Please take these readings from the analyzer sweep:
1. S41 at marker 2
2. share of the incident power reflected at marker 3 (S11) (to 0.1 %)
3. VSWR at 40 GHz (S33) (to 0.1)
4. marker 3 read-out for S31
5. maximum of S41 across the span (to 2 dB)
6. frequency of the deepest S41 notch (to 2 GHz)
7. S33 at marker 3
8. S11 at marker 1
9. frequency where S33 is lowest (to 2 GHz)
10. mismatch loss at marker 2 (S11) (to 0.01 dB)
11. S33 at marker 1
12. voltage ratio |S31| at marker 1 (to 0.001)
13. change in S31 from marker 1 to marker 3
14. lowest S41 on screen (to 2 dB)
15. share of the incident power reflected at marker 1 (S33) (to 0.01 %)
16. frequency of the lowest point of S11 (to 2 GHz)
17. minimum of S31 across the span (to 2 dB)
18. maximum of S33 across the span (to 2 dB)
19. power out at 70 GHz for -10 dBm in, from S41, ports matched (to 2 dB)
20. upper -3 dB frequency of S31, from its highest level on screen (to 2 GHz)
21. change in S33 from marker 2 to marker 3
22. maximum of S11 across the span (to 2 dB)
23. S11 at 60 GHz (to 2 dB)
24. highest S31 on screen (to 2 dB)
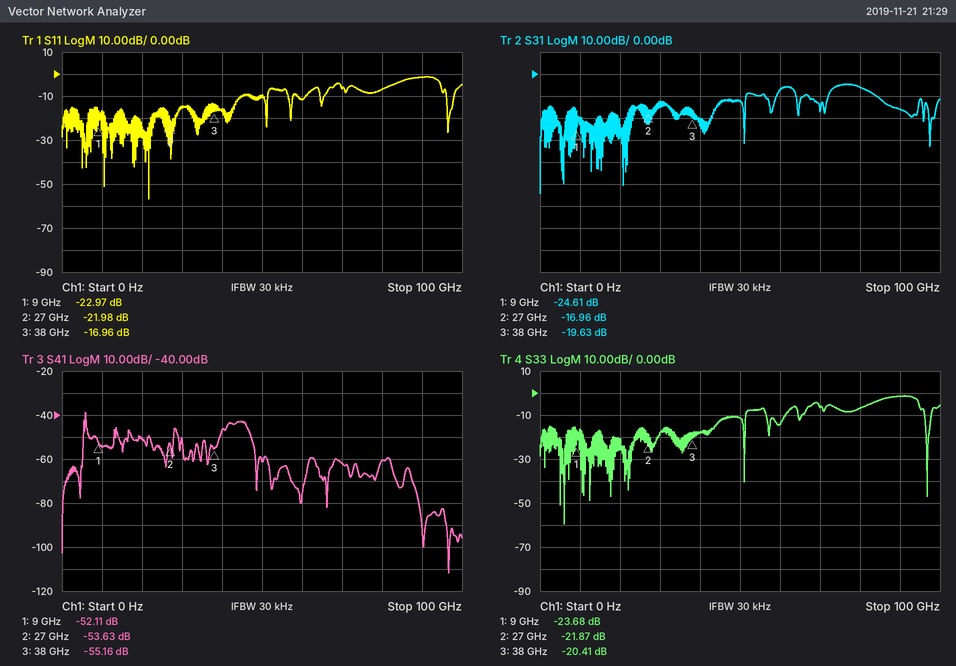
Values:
-53.63 dB
2.0 %
1.3
-19.63 dB
-38 dB
96 GHz
-20.41 dB
-22.97 dB
6 GHz
0.03 dB
-23.68 dB
0.059
4.98 dB
-112 dB
0.43 %
22 GHz
-54 dB
-2 dB
-72 dBm
82 GHz
1.46 dB
-2 dB
-12 dB
-4 dB
